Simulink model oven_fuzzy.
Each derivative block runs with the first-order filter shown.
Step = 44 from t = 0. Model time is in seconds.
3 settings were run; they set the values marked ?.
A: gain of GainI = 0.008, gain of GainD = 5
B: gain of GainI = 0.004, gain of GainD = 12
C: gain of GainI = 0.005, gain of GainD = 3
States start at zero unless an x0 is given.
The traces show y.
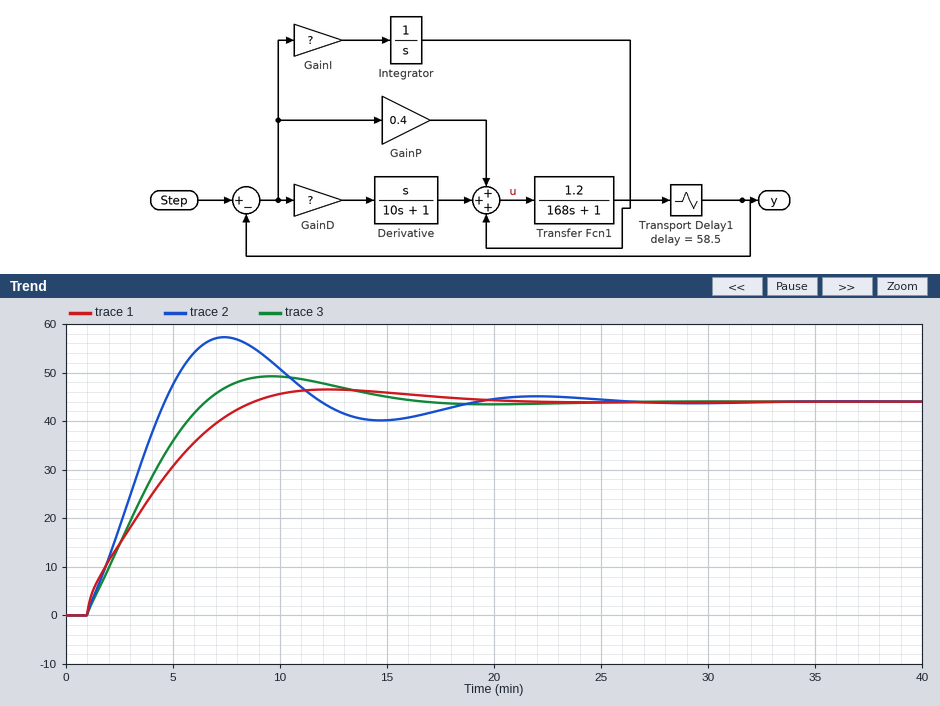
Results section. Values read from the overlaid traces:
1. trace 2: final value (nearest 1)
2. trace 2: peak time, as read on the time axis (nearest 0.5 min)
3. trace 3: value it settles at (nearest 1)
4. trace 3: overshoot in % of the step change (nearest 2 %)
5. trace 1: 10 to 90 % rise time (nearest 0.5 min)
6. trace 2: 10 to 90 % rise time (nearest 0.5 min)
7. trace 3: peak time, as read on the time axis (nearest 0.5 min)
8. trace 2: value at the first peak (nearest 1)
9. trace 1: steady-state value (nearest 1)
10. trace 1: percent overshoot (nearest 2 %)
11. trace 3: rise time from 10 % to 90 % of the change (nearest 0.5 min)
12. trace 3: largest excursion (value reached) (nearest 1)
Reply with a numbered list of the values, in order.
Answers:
1. 44
2. 7.5 min
3. 44
4. 12 %
5. 6.0 min
6. 3.0 min
7. 9.5 min
8. 57
9. 44
10. 6 %
11. 4.0 min
12. 49
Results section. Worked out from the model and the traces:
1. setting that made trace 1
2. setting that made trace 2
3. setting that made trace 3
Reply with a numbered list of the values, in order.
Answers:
1. B
2. A
3. C
